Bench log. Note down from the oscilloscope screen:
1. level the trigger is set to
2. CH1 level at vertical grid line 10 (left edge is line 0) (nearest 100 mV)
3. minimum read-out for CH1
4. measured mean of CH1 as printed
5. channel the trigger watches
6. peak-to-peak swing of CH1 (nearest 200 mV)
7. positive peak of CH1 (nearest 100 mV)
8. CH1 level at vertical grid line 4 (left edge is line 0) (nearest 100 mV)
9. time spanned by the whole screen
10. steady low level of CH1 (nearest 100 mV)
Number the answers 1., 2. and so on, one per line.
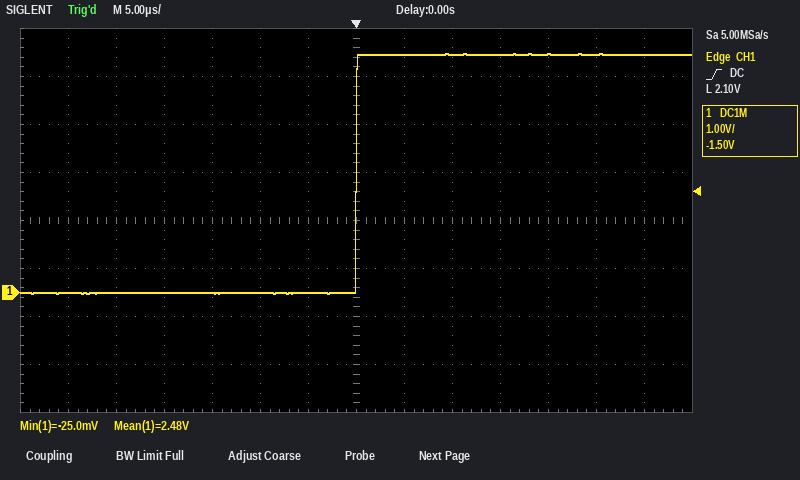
1. 2.10 V
2. 5.0 V
3. -25.0 mV
4. 2.48 V
5. CH1
6. 5.0 V
7. 5.0 V
8. 0.0 V
9. 70 µs
10. 0.0 V
